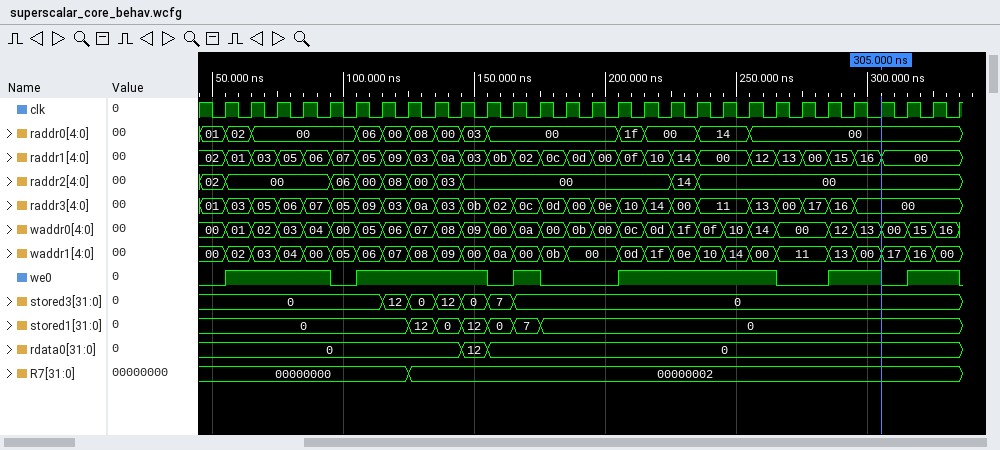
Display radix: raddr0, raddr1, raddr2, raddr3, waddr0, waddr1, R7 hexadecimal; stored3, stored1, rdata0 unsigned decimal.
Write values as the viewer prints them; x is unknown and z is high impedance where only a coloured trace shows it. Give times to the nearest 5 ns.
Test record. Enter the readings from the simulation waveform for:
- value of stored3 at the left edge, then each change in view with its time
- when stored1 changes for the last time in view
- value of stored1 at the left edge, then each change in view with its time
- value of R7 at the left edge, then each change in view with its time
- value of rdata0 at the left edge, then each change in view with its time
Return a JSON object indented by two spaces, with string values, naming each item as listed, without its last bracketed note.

{
  "value of stored3 at the left edge, then each change in view with its time": "0, 12 at 115 ns, 0 at 125 ns, 12 at 135 ns, 0 at 145 ns, 7 at 155 ns, 0 at 165 ns",
  "when stored1 changes for the last time in view": "175 ns",
  "value of stored1 at the left edge, then each change in view with its time": "0, 12 at 125 ns, 0 at 135 ns, 12 at 145 ns, 0 at 155 ns, 7 at 165 ns, 0 at 175 ns",
  "value of R7 at the left edge, then each change in view with its time": "00000000, 00000002 at 125 ns",
  "value of rdata0 at the left edge, then each change in view with its time": "0, 12 at 145 ns, 0 at 155 ns"
}
